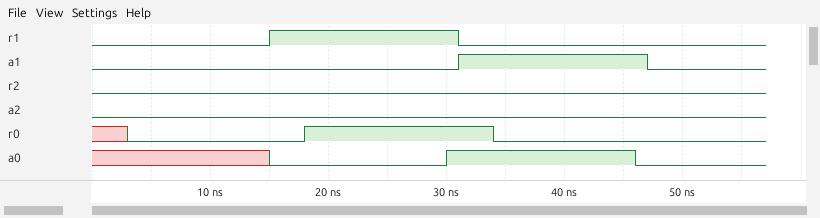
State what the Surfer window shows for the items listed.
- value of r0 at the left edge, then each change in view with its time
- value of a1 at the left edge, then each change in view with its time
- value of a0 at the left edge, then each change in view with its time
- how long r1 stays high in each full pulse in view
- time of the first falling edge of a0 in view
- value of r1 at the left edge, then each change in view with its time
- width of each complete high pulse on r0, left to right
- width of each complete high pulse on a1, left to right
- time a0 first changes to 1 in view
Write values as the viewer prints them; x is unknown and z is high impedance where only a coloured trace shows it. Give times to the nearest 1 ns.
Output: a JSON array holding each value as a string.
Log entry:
["x, 0 at 3 ns, 1 at 18 ns, 0 at 34 ns", "0, 1 at 31 ns, 0 at 47 ns", "x, 0 at 15 ns, 1 at 30 ns, 0 at 46 ns", "16 ns", "46 ns", "0, 1 at 15 ns, 0 at 31 ns", "16 ns", "16 ns", "30 ns"]
